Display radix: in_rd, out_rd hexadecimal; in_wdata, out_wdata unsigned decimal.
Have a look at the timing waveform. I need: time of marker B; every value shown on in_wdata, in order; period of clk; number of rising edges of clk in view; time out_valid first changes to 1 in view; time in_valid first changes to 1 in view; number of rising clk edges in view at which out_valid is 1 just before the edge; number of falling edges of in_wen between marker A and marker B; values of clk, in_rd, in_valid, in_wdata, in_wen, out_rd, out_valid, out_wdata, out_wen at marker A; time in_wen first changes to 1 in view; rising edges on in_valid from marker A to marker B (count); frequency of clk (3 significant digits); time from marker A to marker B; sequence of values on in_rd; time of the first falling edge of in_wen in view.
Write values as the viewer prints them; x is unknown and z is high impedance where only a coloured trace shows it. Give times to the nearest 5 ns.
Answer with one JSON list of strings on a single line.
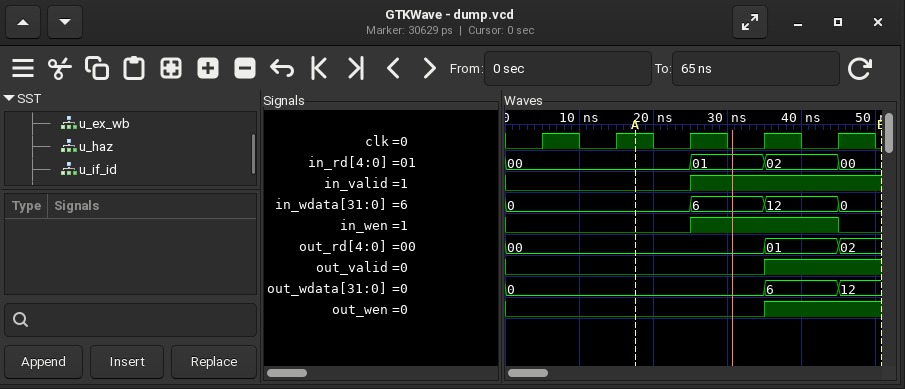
["50 ns", "0, 6, 12, 0", "10 ns", "5", "35 ns", "25 ns", "1", "1", "clk=1, in_rd=00, in_valid=0, in_wdata=0, in_wen=0, out_rd=00, out_valid=0, out_wdata=0, out_wen=0", "25 ns", "1", "100 MHz", "35 ns", "00, 01, 02, 00", "45 ns"]
